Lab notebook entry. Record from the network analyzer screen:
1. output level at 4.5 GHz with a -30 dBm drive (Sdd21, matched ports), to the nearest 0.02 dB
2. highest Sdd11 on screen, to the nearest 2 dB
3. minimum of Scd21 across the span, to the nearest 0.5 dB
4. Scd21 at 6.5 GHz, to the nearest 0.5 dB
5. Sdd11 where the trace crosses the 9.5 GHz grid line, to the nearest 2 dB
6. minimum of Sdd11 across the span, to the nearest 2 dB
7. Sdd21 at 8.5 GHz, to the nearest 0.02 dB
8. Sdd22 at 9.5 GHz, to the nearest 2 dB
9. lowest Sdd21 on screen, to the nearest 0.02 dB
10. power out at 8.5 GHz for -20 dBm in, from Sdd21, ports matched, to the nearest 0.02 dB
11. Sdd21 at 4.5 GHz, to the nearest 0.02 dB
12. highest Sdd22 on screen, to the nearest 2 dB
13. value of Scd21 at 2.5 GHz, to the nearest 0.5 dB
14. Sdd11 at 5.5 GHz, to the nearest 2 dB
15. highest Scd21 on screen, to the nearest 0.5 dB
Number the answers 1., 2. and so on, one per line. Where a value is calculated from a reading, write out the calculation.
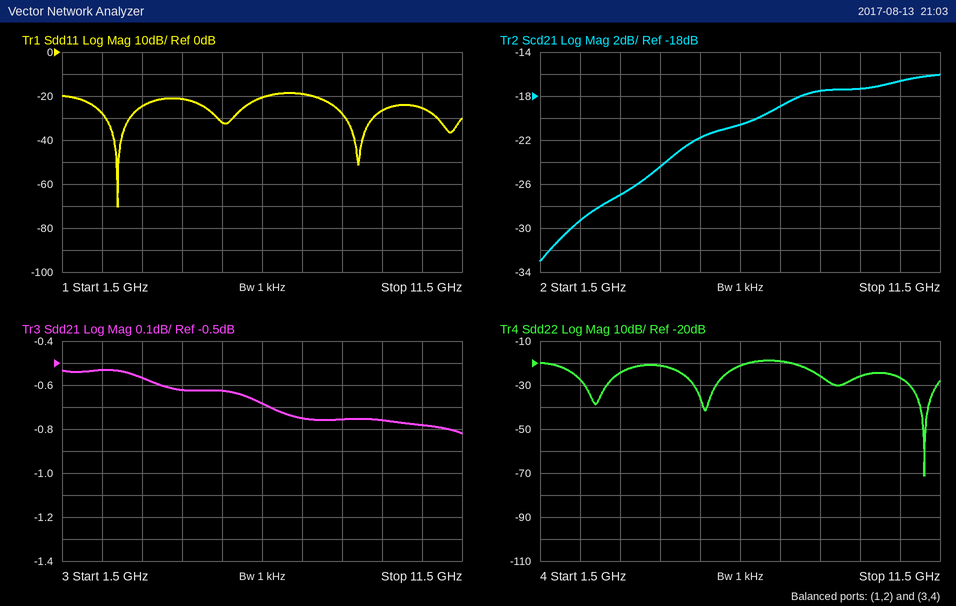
1. -30 dBm + (-0.62 dB) = -30.62 dBm
2. -18 dB
3. -33.0 dB
4. -20.5 dB
5. -26 dB
6. -70 dB
7. -0.76 dB
8. -26 dB
9. -0.82 dB
10. -20 dBm + (-0.76 dB) = -20.76 dBm
11. -0.62 dB
12. -18 dB
13. -29.5 dB
14. -32 dB
15. -16.0 dB
